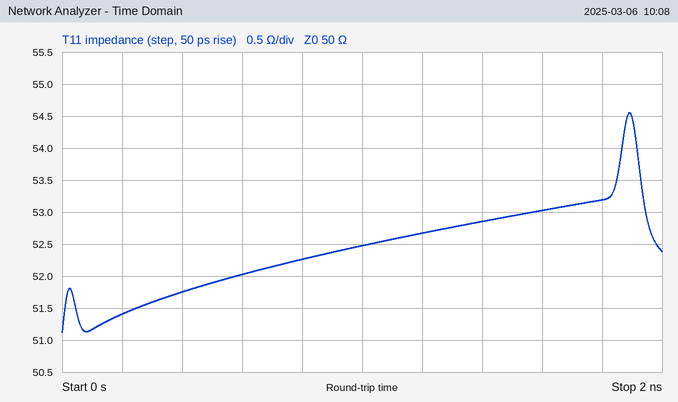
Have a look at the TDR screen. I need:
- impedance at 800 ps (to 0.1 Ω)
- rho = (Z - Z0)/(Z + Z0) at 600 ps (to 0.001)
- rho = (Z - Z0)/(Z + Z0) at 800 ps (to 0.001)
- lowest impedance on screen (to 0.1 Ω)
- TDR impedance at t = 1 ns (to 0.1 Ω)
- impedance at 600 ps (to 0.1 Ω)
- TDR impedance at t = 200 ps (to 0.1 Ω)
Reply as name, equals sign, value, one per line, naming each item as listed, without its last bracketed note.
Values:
impedance at 800 ps = 52.3 Ω
rho = (Z - Z0)/(Z + Z0) at 600 ps = +0.020
rho = (Z - Z0)/(Z + Z0) at 800 ps = +0.022
lowest impedance on screen = 51.1 Ω
TDR impedance at t = 1 ns = 52.5 Ω
impedance at 600 ps = 52.0 Ω
TDR impedance at t = 200 ps = 51.4 Ω
